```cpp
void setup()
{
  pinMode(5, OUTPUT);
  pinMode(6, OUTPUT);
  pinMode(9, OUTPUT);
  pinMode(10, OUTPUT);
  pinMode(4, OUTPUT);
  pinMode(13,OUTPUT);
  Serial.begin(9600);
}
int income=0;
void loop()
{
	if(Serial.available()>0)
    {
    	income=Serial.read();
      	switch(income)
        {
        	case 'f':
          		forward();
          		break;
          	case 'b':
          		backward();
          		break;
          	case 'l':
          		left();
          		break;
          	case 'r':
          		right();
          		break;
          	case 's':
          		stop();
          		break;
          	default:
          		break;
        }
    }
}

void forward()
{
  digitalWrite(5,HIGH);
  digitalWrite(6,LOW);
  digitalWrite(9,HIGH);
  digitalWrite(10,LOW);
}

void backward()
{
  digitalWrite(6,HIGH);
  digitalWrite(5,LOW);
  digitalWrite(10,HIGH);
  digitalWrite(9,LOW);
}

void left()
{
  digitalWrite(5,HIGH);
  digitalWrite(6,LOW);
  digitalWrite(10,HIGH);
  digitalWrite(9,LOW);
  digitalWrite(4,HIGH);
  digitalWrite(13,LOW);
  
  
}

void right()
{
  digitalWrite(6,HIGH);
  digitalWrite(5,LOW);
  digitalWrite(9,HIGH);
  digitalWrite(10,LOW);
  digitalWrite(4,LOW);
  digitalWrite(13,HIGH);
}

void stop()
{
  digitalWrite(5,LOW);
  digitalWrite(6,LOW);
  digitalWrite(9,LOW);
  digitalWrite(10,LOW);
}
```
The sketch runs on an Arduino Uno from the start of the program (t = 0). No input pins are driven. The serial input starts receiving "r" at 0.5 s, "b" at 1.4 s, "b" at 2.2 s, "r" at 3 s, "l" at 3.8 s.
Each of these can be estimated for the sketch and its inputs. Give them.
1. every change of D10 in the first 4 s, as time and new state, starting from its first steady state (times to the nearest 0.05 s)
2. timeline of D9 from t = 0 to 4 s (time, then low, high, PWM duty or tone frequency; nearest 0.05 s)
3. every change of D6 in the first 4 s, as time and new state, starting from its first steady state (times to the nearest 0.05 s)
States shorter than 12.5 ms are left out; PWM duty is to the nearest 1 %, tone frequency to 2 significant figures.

0 s low; 1.4 s high; 3 s low; 3.8 s high
0 s low; 0.5 s high; 1.4 s low; 3 s high; 3.8 s low
0 s low; 0.5 s high; 3.8 s low
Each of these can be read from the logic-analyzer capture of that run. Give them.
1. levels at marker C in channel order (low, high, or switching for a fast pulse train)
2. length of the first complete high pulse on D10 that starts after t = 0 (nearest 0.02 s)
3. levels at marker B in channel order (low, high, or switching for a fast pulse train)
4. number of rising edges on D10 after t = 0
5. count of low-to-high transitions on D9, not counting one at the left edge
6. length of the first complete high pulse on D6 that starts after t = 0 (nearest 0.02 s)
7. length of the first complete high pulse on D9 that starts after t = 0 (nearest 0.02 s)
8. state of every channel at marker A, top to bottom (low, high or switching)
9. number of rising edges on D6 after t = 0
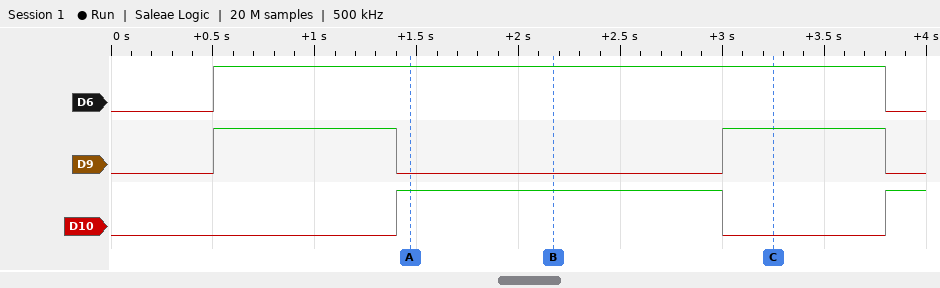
D6 high, D9 high, D10 low
1.60 s
D6 high, D9 low, D10 high
2
2
3.30 s
0.90 s
D6 high, D9 low, D10 high
1
